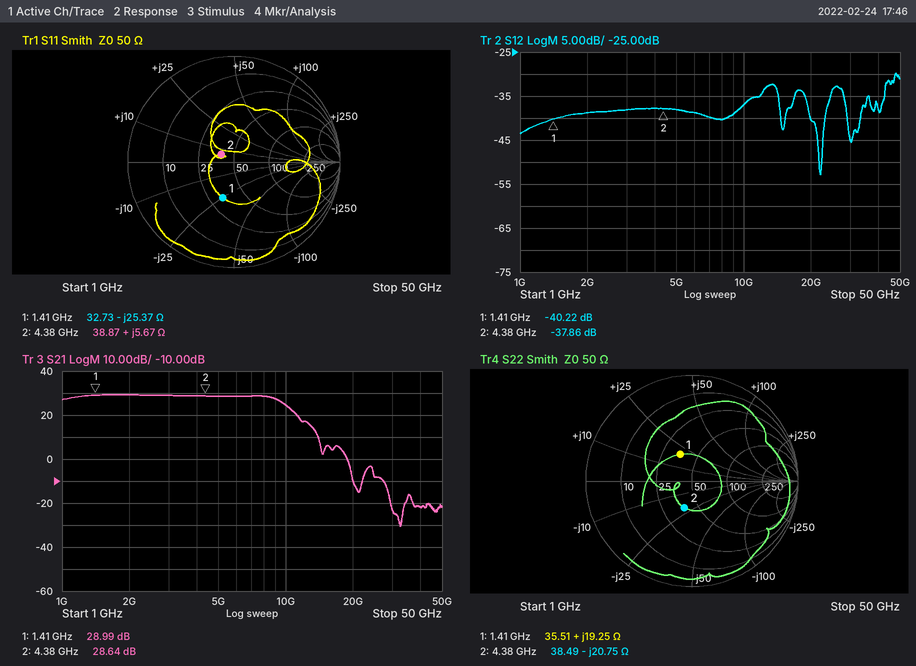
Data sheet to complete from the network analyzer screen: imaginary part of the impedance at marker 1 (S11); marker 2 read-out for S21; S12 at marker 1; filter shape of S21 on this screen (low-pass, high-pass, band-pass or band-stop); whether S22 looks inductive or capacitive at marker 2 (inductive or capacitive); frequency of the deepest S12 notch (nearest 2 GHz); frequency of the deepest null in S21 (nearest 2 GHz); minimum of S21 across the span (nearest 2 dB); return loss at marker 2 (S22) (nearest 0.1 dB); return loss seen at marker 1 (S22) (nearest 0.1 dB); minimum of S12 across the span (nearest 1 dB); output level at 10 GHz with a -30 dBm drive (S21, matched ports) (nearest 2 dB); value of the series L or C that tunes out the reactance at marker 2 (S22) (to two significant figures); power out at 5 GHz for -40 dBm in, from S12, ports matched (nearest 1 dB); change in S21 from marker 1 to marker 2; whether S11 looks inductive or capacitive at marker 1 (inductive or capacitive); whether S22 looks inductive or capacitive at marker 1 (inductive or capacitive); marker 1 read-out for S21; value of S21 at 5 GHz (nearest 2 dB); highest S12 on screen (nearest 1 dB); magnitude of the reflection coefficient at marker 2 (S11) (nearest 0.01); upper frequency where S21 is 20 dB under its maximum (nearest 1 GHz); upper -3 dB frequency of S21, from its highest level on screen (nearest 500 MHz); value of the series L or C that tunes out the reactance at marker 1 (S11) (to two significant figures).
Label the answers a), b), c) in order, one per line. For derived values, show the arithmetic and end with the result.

a) -25.37 Ω
b) 28.64 dB
c) -40.22 dB
d) low-pass
e) capacitive
f) 22 GHz
g) 32 GHz
h) -30 dB
i) 11.7 dB
j) 11.2 dB
k) -53 dB
l) -30 dBm + (24 dB) = -6 dBm
m) L = 20.75 Ω/(2π × 4.38 GHz) ≈ 754 pH, so 750 pH to two significant figures
n) -40 dBm + (-38 dB) = -78 dBm
o) 28.64 − (28.99) = -0.35 dB
p) capacitive
q) inductive
r) 28.99 dB
s) 28 dB
t) -30 dB
u) 0.14
v) 14 GHz
w) 9.5 GHz
x) L = 25.37 Ω/(2π × 1.41 GHz) ≈ 2.9 nH
